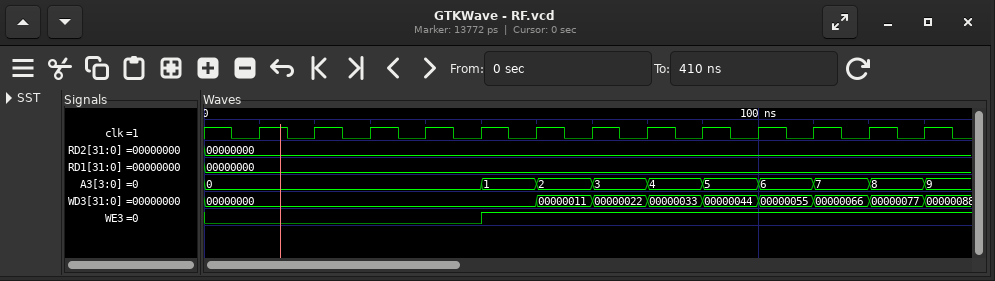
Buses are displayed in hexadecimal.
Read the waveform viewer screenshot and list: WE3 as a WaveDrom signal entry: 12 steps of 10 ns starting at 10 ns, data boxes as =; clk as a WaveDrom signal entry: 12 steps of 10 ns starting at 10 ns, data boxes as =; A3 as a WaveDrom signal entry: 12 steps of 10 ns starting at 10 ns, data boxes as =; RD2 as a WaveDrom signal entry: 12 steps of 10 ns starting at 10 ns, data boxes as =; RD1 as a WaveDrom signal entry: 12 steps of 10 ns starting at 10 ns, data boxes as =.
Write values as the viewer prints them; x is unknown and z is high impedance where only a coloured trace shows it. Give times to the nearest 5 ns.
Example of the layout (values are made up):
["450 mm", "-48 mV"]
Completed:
["{name: 'WE3', wave: '0...1.......'}", "{name: 'clk', wave: 'p...........'}", "{name: 'A3', wave: '=...========', data: '0 1 2 3 4 5 6 7 8'}", "{name: 'RD2', wave: '=...........', data: '00000000'}", "{name: 'RD1', wave: '=...........', data: '00000000'}"]
